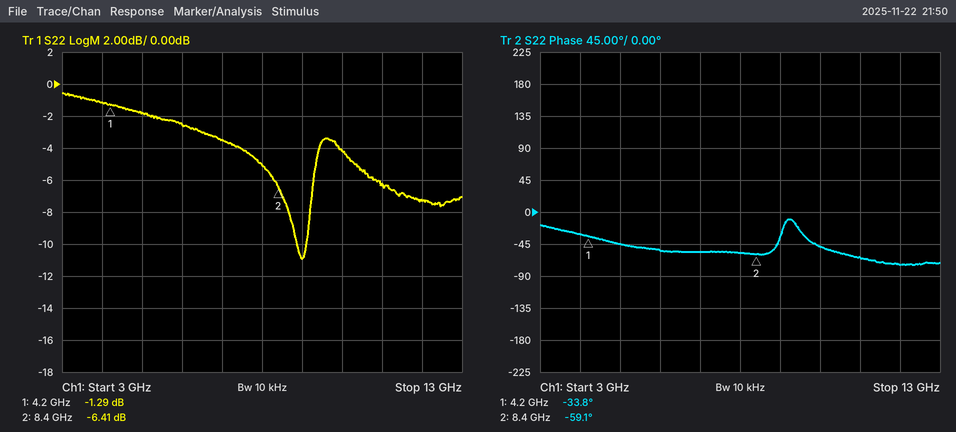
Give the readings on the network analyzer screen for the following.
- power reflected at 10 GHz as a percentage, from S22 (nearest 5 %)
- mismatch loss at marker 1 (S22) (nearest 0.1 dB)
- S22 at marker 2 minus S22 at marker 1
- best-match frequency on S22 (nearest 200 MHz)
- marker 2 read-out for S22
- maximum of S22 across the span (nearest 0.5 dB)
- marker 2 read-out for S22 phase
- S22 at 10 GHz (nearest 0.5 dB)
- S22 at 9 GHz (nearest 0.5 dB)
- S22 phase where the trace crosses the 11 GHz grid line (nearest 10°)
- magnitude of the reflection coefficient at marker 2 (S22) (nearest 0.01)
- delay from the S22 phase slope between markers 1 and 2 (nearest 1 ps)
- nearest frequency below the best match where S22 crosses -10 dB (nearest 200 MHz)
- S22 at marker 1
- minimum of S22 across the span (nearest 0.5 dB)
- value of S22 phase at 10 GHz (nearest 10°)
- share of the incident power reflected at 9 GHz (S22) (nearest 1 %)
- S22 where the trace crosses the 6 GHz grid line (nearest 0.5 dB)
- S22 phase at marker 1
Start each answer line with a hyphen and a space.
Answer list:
- 40 %
- 5.9 dB
- -5.12 dB
- 9.0 GHz
- -6.41 dB
- -0.5 dB
- -59.1°
- -4.0 dB
- -11.0 dB
- -60°
- 0.48
- 17 ps
- 8.8 GHz
- -1.29 dB
- -11.0 dB
- -50°
- 8 %
- -2.5 dB
- -33.8°
